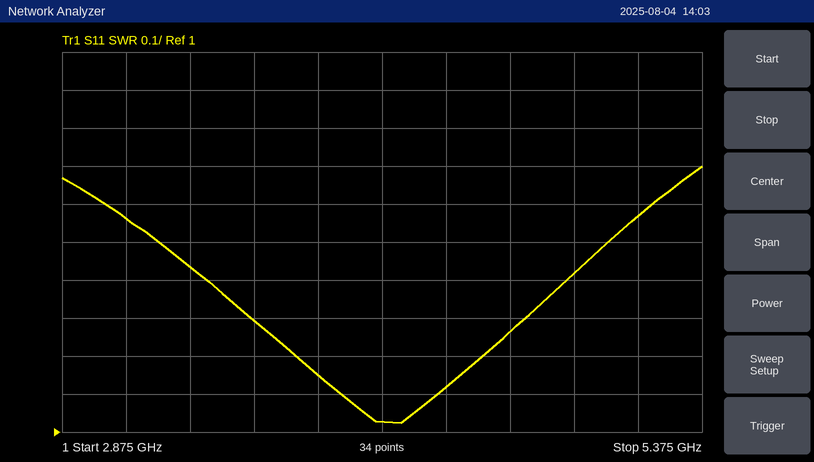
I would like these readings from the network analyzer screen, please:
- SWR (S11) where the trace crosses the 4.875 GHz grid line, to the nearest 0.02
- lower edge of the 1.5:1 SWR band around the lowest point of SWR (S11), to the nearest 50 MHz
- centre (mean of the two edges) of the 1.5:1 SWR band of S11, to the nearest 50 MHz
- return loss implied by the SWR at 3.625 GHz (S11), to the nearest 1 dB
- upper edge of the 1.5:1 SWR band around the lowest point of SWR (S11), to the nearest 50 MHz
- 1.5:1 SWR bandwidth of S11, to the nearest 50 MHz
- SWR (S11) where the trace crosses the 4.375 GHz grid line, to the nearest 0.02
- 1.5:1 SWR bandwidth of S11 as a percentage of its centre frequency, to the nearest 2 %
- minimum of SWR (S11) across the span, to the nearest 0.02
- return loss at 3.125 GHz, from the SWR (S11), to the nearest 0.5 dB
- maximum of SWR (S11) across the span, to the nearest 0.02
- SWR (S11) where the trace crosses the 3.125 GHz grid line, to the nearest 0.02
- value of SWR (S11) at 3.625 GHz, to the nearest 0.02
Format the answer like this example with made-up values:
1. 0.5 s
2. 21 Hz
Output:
1. 1.42
2. 3.25 GHz
3. 4.15 GHz
4. 18 dB
5. 5.00 GHz
6. 1.75 GHz
7. 1.12
8. 42 %
9. 1.02
10. 13.0 dB
11. 1.70
12. 1.56
13. 1.30
